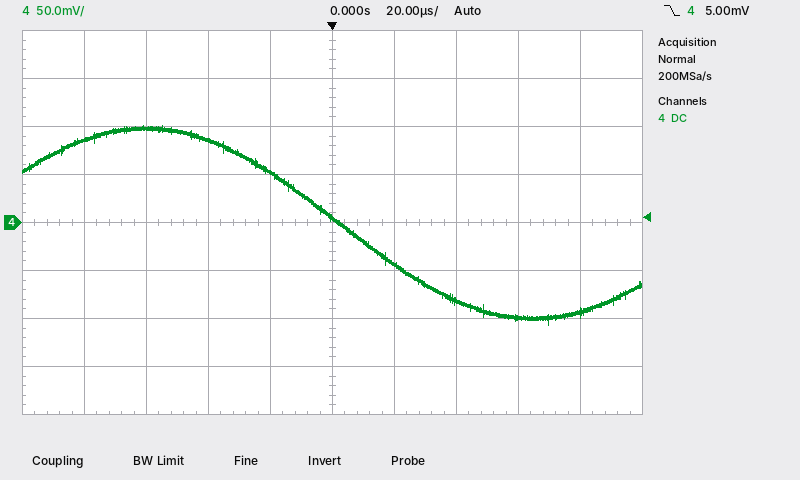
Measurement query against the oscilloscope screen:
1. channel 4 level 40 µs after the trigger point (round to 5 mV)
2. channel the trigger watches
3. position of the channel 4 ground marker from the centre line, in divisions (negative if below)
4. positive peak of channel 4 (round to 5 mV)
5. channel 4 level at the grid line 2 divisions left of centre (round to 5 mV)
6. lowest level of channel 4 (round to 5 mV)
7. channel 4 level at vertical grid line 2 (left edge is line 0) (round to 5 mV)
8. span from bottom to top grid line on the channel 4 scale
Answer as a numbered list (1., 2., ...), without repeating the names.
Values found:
1. -80 mV
2. channel 4
3. 0.0 div
4. 100 mV
5. 85 mV
6. -105 mV
7. 100 mV
8. 400 mV
